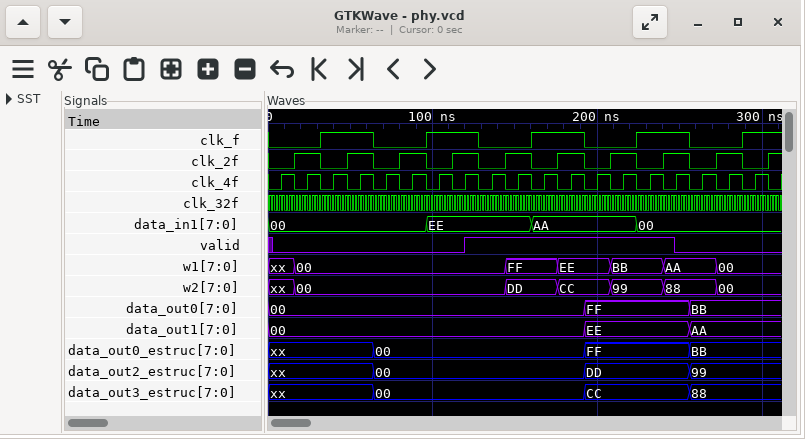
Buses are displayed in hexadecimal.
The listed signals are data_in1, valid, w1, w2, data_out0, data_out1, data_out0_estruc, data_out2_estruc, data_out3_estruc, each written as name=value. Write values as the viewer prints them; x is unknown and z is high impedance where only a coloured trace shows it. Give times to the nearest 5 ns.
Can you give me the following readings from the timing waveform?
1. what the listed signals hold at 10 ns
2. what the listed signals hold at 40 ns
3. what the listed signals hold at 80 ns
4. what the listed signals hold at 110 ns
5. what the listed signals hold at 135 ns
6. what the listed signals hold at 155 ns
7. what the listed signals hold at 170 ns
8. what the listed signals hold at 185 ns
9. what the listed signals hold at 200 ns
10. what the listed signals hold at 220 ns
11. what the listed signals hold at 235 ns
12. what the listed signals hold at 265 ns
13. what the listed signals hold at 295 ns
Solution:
data_in1=00, valid=0, w1=xx, w2=xx, data_out0=00, data_out1=00, data_out0_estruc=xx, data_out2_estruc=xx, data_out3_estruc=xx
data_in1=00, valid=0, w1=00, w2=00, data_out0=00, data_out1=00, data_out0_estruc=xx, data_out2_estruc=xx, data_out3_estruc=xx
data_in1=00, valid=0, w1=00, w2=00, data_out0=00, data_out1=00, data_out0_estruc=00, data_out2_estruc=00, data_out3_estruc=00
data_in1=EE, valid=0, w1=00, w2=00, data_out0=00, data_out1=00, data_out0_estruc=00, data_out2_estruc=00, data_out3_estruc=00
data_in1=EE, valid=1, w1=00, w2=00, data_out0=00, data_out1=00, data_out0_estruc=00, data_out2_estruc=00, data_out3_estruc=00
data_in1=EE, valid=1, w1=FF, w2=DD, data_out0=00, data_out1=00, data_out0_estruc=00, data_out2_estruc=00, data_out3_estruc=00
data_in1=AA, valid=1, w1=FF, w2=DD, data_out0=00, data_out1=00, data_out0_estruc=00, data_out2_estruc=00, data_out3_estruc=00
data_in1=AA, valid=1, w1=EE, w2=CC, data_out0=00, data_out1=00, data_out0_estruc=00, data_out2_estruc=00, data_out3_estruc=00
data_in1=AA, valid=1, w1=EE, w2=CC, data_out0=FF, data_out1=EE, data_out0_estruc=FF, data_out2_estruc=DD, data_out3_estruc=CC
data_in1=AA, valid=1, w1=BB, w2=99, data_out0=FF, data_out1=EE, data_out0_estruc=FF, data_out2_estruc=DD, data_out3_estruc=CC
data_in1=00, valid=1, w1=BB, w2=99, data_out0=FF, data_out1=EE, data_out0_estruc=FF, data_out2_estruc=DD, data_out3_estruc=CC
data_in1=00, valid=0, w1=AA, w2=88, data_out0=BB, data_out1=AA, data_out0_estruc=BB, data_out2_estruc=99, data_out3_estruc=88
data_in1=00, valid=0, w1=00, w2=00, data_out0=BB, data_out1=AA, data_out0_estruc=BB, data_out2_estruc=99, data_out3_estruc=88
